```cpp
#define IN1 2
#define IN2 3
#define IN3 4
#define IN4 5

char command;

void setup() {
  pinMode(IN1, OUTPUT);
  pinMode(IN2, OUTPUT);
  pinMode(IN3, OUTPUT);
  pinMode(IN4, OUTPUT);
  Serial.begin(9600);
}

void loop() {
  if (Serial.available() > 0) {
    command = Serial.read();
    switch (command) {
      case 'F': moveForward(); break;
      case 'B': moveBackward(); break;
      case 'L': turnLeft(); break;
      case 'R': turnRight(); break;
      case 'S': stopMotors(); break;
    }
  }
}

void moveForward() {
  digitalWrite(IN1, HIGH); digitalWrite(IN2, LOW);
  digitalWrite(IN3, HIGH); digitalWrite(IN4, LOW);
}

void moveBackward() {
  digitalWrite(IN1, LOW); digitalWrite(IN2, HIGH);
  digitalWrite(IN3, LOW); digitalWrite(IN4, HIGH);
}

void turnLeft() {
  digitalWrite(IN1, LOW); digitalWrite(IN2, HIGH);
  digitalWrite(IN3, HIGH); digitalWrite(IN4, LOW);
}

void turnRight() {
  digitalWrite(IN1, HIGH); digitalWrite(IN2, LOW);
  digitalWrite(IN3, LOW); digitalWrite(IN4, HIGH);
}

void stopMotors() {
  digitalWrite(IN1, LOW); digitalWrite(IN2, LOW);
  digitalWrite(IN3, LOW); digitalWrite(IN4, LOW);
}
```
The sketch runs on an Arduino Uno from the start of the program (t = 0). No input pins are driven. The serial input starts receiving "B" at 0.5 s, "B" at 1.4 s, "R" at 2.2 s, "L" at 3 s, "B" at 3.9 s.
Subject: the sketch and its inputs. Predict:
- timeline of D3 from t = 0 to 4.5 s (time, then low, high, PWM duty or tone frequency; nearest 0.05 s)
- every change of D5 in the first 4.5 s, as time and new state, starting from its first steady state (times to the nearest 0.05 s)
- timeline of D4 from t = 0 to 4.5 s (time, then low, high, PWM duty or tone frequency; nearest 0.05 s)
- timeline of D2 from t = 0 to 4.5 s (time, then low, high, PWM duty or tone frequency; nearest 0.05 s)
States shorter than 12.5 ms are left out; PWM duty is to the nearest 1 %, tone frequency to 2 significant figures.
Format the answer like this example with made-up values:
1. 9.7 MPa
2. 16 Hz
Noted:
1. 0 s low; 0.5 s high; 2.2 s low; 3 s high
2. 0 s low; 0.5 s high; 3 s low; 3.9 s high
3. 0 s low; 3 s high; 3.9 s low
4. 0 s low; 2.2 s high; 3 s low
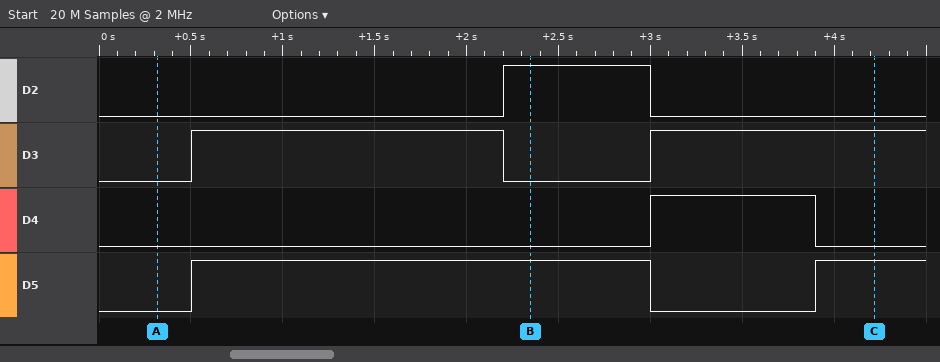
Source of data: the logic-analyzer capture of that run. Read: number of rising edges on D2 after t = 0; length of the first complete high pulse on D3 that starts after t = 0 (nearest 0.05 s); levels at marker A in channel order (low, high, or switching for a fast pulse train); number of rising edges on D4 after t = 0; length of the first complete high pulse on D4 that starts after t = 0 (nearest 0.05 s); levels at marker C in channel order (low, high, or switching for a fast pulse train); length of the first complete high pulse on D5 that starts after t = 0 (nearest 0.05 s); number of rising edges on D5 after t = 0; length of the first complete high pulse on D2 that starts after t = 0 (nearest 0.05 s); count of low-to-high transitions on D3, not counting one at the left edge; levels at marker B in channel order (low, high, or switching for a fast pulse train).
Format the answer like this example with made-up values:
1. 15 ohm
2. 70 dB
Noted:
1. 1
2. 1.70 s
3. D2 low, D3 low, D4 low, D5 low
4. 1
5. 0.90 s
6. D2 low, D3 high, D4 low, D5 high
7. 2.50 s
8. 2
9. 0.80 s
10. 2
11. D2 high, D3 low, D4 low, D5 high
